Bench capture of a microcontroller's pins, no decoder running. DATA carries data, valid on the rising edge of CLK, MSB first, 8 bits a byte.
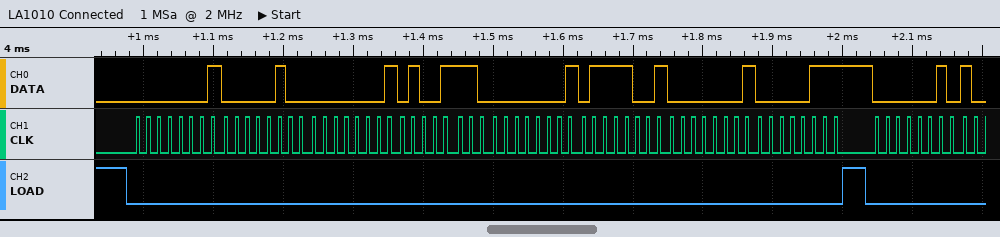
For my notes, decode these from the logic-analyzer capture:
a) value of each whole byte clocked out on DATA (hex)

01 04 01 4E 01 79 01 07 02
